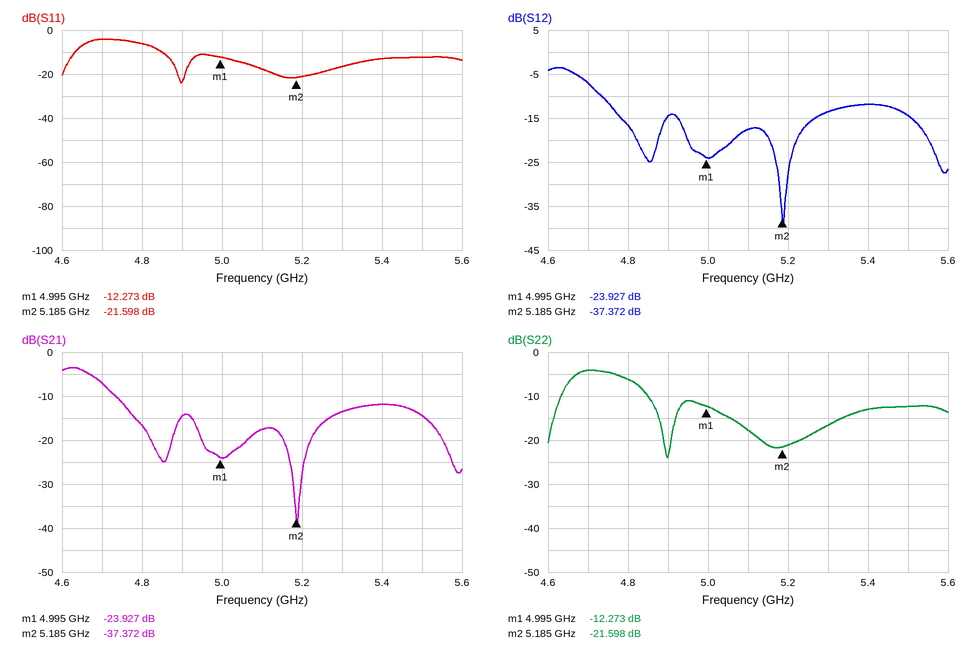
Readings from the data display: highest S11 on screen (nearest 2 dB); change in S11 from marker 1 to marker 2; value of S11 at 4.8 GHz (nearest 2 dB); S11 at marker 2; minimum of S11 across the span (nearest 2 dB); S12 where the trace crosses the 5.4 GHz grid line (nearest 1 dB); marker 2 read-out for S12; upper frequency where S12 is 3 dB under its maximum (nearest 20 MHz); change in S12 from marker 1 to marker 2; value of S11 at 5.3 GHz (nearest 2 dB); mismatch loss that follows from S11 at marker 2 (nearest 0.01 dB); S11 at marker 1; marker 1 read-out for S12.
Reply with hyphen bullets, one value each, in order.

- -4 dB
- -9.325 dB
- -6 dB
- -21.598 dB
- -24 dB
- -12 dB
- -37.372 dB
- 4.70 GHz
- -13.445 dB
- -16 dB
- 0.03 dB
- -12.273 dB
- -23.927 dB
